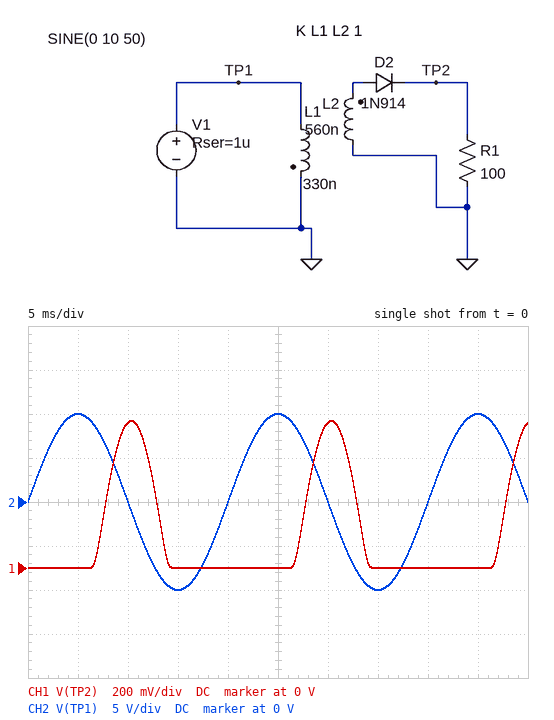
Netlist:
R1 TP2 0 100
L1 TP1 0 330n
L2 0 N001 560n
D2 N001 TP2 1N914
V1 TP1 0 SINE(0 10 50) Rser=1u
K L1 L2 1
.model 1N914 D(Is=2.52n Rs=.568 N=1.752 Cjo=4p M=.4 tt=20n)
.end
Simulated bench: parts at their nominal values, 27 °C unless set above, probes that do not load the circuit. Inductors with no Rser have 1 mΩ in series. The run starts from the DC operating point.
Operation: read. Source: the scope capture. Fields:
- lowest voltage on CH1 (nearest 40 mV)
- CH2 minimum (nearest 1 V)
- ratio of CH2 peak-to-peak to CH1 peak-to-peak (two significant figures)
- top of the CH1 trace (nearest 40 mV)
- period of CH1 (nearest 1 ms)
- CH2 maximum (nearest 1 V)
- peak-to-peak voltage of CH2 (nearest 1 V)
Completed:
0 V
-10 V
30
680 mV
20 ms
10 V
20 V
